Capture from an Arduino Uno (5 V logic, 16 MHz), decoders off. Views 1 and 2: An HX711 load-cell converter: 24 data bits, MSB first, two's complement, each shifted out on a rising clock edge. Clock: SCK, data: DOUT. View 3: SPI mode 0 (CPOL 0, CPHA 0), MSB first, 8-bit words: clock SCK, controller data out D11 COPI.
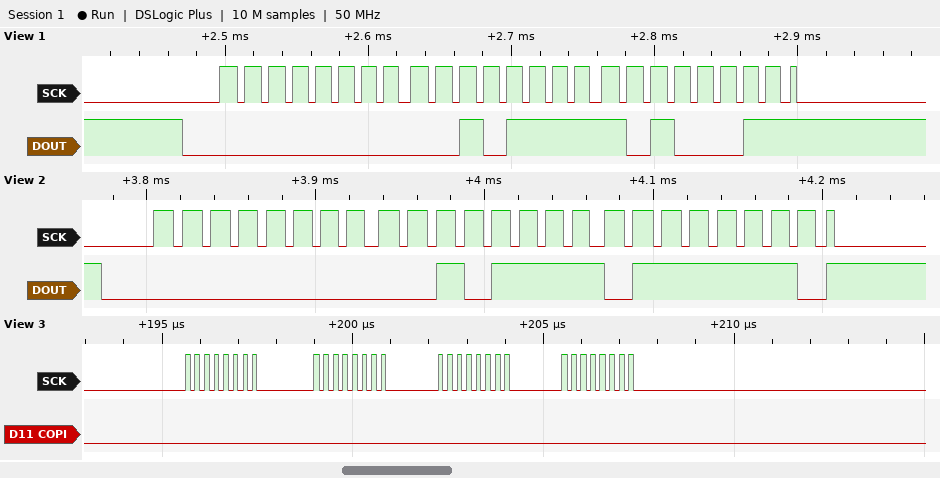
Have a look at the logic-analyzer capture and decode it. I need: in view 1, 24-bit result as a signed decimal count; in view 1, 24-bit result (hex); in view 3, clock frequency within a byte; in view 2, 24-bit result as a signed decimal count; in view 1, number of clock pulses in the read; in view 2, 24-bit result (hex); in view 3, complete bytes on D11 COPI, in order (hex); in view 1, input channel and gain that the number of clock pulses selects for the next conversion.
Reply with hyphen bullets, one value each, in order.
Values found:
- 12195
- 0x002FA3
- 4 MHz
- 12158
- 25
- 0x002F7E
- 0x00 0x00 0x00 0x00
- channel A, gain 128
